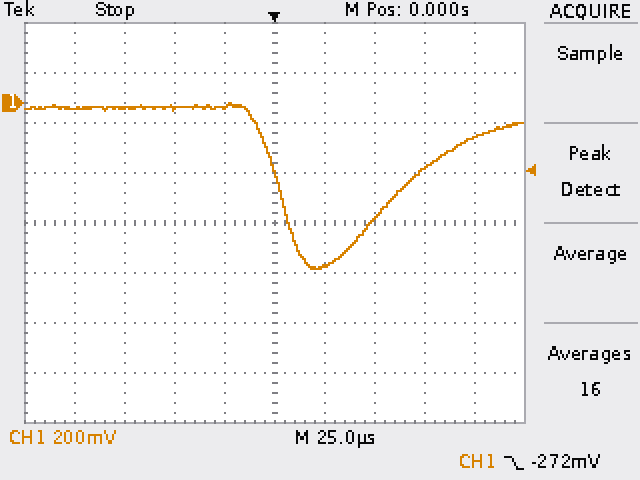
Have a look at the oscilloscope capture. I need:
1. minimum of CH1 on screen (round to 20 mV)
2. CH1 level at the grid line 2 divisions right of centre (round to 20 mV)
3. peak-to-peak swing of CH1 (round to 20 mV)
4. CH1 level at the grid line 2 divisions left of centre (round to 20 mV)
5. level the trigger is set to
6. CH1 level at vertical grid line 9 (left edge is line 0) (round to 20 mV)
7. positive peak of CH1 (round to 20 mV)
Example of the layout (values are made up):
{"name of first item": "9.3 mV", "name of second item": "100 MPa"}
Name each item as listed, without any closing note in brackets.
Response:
{"minimum of CH1 on screen": "-660 mV", "CH1 level at the grid line 2 divisions right of centre": "-460 mV", "peak-to-peak swing of CH1": "660 mV", "CH1 level at the grid line 2 divisions left of centre": "-20 mV", "level the trigger is set to": "-272 mV", "CH1 level at vertical grid line 9 (left edge is line 0)": "-140 mV", "positive peak of CH1": "0 mV"}
